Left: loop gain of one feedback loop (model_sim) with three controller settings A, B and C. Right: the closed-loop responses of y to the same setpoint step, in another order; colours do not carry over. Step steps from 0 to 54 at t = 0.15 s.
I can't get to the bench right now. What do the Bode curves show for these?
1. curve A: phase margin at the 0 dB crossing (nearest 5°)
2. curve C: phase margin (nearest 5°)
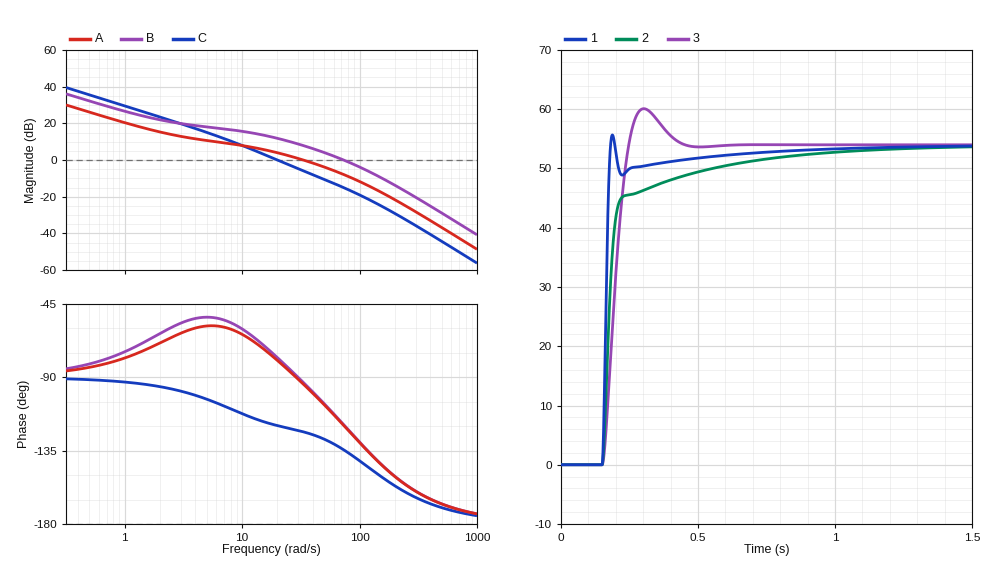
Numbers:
85°
60°
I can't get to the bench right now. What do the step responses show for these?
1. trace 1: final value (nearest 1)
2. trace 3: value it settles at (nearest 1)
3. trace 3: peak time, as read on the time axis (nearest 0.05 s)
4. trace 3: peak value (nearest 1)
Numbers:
54
54
0.30 s
60
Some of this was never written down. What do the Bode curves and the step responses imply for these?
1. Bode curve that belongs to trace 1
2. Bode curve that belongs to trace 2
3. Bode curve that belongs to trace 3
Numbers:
B
A
C
